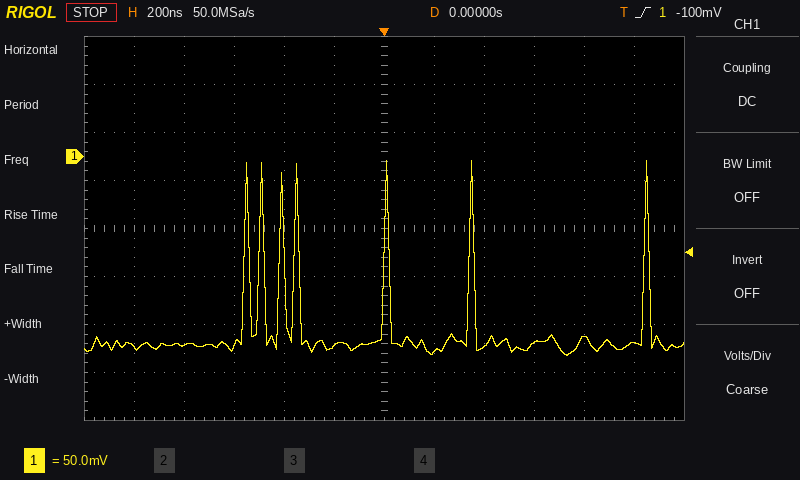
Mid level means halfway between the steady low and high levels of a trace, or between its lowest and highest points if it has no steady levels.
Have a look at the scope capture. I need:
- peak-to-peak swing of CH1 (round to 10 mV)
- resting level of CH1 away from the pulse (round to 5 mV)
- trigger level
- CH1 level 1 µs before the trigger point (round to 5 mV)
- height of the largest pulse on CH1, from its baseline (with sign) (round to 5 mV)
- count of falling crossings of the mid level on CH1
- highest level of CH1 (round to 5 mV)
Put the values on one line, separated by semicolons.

200 mV; -195 mV; -100 mV; -200 mV; +190 mV; 7; -5 mV
